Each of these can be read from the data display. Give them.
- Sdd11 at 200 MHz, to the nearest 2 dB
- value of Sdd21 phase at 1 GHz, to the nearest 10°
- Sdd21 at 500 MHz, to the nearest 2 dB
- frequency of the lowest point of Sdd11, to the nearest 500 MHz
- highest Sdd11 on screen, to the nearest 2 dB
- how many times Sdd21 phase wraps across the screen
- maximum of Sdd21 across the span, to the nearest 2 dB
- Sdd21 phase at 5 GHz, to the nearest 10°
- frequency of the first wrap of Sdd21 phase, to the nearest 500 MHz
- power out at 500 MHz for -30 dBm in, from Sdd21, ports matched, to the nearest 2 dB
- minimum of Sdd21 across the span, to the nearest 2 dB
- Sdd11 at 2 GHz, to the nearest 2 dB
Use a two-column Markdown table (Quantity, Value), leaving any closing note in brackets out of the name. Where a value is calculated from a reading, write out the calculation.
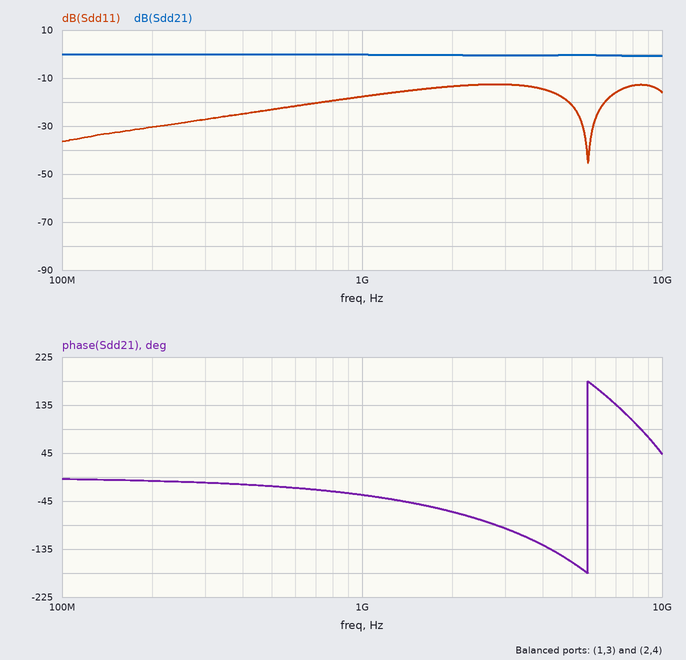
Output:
| Quantity | Value |
|---|---|
| Sdd11 at 200 MHz, to the nearest 2 dB | -30 dB |
| value of Sdd21 phase at 1 GHz, to the nearest 10° | -30° |
| Sdd21 at 500 MHz, to the nearest 2 dB | 0 dB |
| frequency of the lowest point of Sdd11, to the nearest 500 MHz | 5.5 GHz |
| highest Sdd11 on screen, to the nearest 2 dB | -12 dB |
| how many times Sdd21 phase wraps across the screen | 1 |
| maximum of Sdd21 across the span, to the nearest 2 dB | 0 dB |
| Sdd21 phase at 5 GHz, to the nearest 10° | -160° |
| frequency of the first wrap of Sdd21 phase, to the nearest 500 MHz | 5.5 GHz |
| power out at 500 MHz for -30 dBm in, from Sdd21, ports matched, to the nearest 2 dB | -30 dBm + (0 dB) = -30 dBm |
| minimum of Sdd21 across the span, to the nearest 2 dB | 0 dB |
| Sdd11 at 2 GHz, to the nearest 2 dB | -14 dB |
